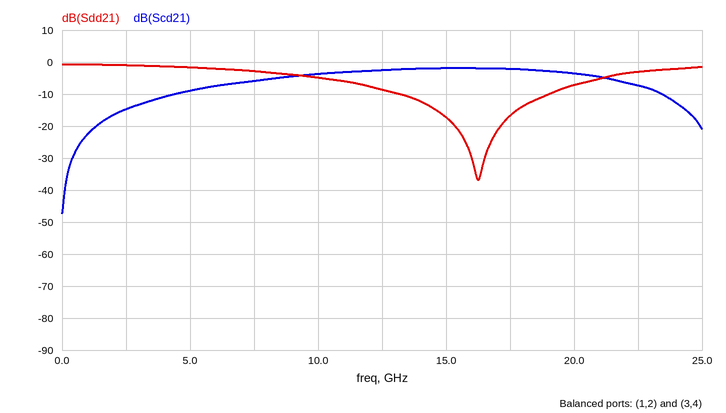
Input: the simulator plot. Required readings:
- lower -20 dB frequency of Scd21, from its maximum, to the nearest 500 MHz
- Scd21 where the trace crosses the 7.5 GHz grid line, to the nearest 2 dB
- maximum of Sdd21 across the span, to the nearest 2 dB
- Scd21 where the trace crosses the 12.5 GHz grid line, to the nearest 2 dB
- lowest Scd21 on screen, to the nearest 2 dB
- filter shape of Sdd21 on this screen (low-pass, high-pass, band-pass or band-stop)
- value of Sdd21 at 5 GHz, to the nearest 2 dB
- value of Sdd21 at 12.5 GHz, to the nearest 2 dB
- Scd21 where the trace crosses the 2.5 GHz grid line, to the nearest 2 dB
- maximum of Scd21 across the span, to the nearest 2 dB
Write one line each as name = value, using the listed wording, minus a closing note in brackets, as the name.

lower -20 dB frequency of Scd21, from its maximum, to the nearest 500 MHz = 1.0 GHz
Scd21 where the trace crosses the 7.5 GHz grid line, to the nearest 2 dB = -6 dB
maximum of Sdd21 across the span, to the nearest 2 dB = 0 dB
Scd21 where the trace crosses the 12.5 GHz grid line, to the nearest 2 dB = -2 dB
lowest Scd21 on screen, to the nearest 2 dB = -48 dB
filter shape of Sdd21 on this screen = band-stop
value of Sdd21 at 5 GHz, to the nearest 2 dB = -2 dB
value of Sdd21 at 12.5 GHz, to the nearest 2 dB = -8 dB
Scd21 where the trace crosses the 2.5 GHz grid line, to the nearest 2 dB = -14 dB
maximum of Scd21 across the span, to the nearest 2 dB = -2 dB
